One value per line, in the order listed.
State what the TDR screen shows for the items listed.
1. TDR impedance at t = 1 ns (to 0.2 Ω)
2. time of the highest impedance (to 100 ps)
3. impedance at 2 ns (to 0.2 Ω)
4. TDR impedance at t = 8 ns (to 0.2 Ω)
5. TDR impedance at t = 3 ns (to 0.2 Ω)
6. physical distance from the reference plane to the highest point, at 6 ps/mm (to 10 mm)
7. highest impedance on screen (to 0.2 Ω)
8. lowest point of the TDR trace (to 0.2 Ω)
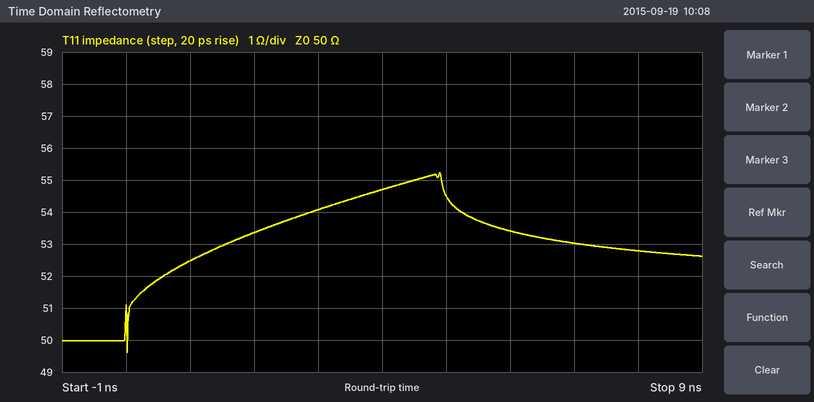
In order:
52.4 Ω
4.9 ns
53.4 Ω
52.8 Ω
54.0 Ω
410 mm
55.2 Ω
49.6 Ω
